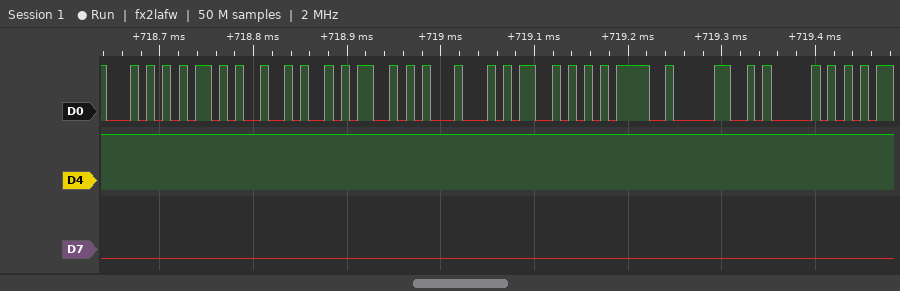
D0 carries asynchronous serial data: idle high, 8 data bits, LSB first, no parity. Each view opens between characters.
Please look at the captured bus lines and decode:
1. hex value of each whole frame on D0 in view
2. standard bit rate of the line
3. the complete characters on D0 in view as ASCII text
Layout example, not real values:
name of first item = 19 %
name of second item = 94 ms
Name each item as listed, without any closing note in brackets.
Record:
hex value of each whole frame on D0 in view = 54, 2B, 4A, 53, 44, 53, 3D, 30, 41
standard bit rate of the line = 115200 baud
the complete characters on D0 in view as ASCII text = "T+JSDS=0A"
